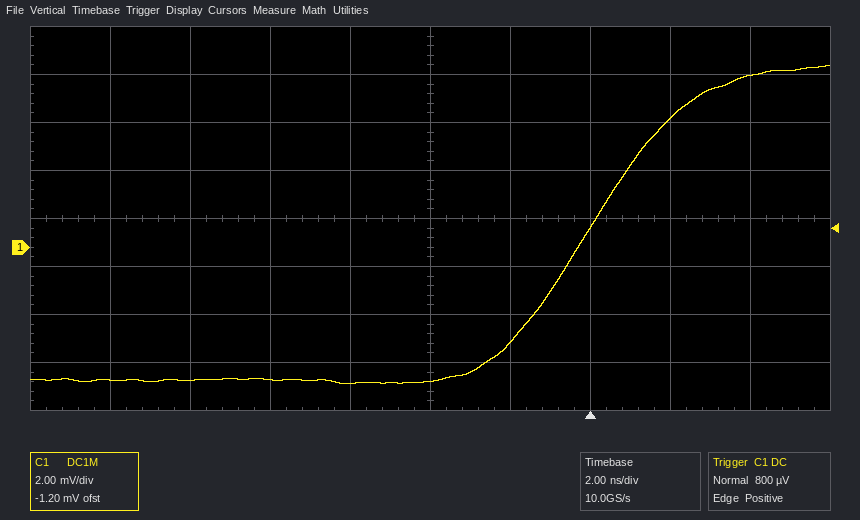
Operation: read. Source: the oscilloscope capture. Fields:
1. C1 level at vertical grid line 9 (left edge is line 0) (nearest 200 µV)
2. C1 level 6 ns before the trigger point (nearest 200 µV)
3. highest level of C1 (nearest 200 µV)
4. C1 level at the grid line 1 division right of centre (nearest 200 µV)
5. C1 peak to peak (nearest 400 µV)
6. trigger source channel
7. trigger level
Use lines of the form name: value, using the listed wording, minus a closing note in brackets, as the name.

C1 level at vertical grid line 9 (left edge is line 0): 7.2 mV
C1 level 6 ns before the trigger point: -5.6 mV
highest level of C1: 7.6 mV
C1 level at the grid line 1 division right of centre: -4.0 mV
C1 peak to peak: 13.2 mV
trigger source channel: C1
trigger level: 800 µV
